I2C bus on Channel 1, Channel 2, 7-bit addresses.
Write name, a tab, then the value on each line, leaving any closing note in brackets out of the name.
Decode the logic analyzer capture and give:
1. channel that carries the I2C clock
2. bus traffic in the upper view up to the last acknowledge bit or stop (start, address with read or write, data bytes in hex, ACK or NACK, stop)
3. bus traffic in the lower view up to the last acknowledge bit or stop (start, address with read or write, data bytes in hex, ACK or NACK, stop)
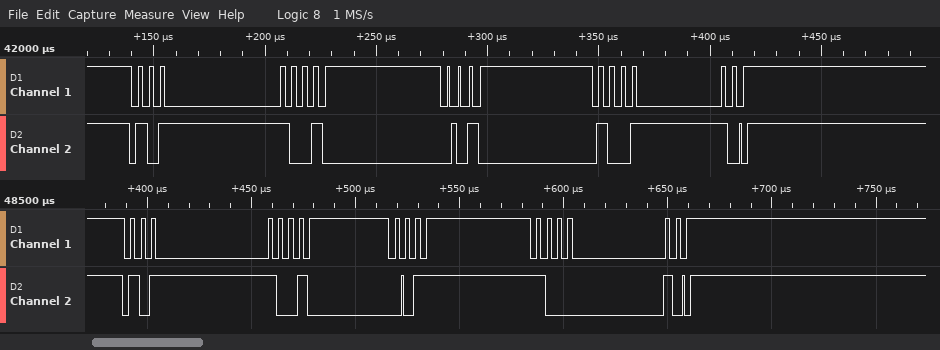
channel that carries the I2C clock	Channel 1
bus traffic in the upper view up to the last acknowledge bit or stop	start, address 59 write ACK, 53 ACK, stop
bus traffic in the lower view up to the last acknowledge bit or stop	start, address 59 write ACK, 71 ACK, stop
